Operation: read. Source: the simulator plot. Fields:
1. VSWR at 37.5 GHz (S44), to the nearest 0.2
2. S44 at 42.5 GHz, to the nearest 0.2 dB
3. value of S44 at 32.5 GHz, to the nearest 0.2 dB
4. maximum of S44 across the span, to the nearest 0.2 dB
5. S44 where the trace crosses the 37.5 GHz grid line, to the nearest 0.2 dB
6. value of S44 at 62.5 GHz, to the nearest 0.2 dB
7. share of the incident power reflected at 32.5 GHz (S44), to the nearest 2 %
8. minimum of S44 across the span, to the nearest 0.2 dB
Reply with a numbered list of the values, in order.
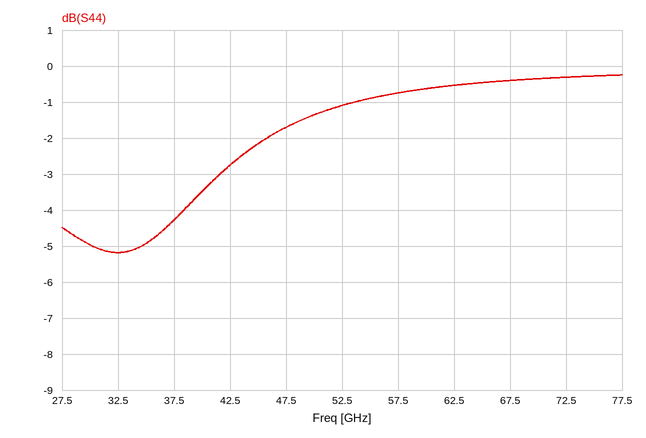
1. 4.2
2. -2.8 dB
3. -5.2 dB
4. -0.2 dB
5. -4.2 dB
6. -0.6 dB
7. 30 %
8. -5.2 dB
